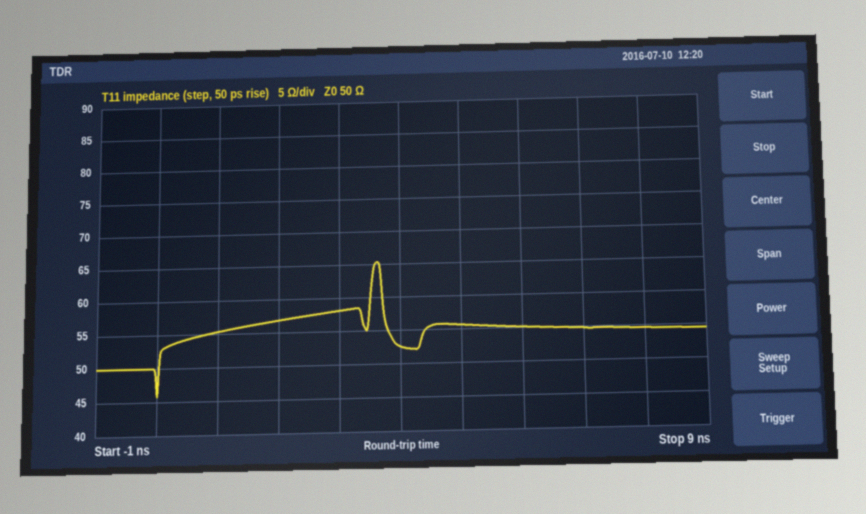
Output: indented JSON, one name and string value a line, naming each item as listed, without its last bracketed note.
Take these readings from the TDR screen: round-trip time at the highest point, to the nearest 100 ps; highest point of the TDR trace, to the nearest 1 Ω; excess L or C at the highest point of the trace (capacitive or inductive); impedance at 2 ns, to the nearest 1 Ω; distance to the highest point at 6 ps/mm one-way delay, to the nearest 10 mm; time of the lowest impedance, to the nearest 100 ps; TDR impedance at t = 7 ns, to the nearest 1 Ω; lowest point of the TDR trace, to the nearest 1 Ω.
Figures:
{
  "round-trip time at the highest point, to the nearest 100 ps": "3.6 ns",
  "highest point of the TDR trace, to the nearest 1 Ω": "65 Ω",
  "excess L or C at the highest point of the trace": "inductive",
  "impedance at 2 ns, to the nearest 1 Ω": "57 Ω",
  "distance to the highest point at 6 ps/mm one-way delay, to the nearest 10 mm": "300 mm",
  "time of the lowest impedance, to the nearest 100 ps": "0.0 ns",
  "TDR impedance at t = 7 ns, to the nearest 1 Ω": "55 Ω",
  "lowest point of the TDR trace, to the nearest 1 Ω": "46 Ω"
}
